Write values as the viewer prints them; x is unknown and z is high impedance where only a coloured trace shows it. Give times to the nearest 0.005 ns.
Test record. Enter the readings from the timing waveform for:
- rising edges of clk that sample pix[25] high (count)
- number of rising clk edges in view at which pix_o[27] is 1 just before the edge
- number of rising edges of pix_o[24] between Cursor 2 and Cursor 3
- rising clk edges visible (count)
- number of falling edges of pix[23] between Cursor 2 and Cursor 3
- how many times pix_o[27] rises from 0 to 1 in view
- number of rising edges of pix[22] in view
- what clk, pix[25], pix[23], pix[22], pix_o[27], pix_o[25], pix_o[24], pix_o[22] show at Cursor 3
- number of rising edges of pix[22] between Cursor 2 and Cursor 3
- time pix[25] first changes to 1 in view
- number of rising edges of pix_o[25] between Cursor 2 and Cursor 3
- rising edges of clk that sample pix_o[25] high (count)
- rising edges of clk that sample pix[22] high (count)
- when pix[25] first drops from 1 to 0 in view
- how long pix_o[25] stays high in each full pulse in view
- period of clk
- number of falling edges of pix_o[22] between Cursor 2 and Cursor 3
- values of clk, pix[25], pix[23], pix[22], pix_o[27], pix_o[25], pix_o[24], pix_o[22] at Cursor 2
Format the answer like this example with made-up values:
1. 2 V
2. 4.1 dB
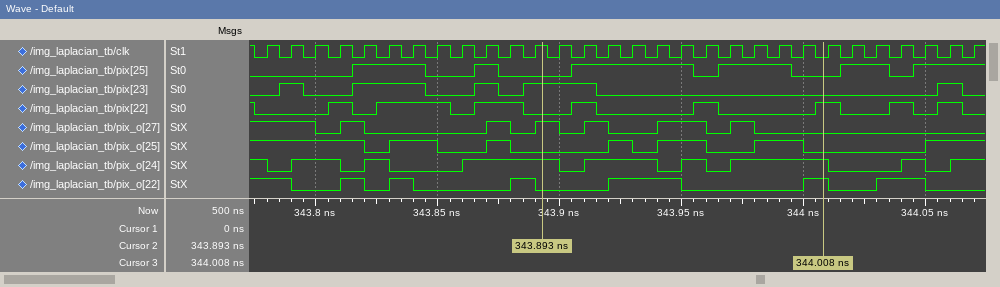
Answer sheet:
1. 17
2. 10
3. 3
4. 30
5. 1
6. 6
7. 8
8. clk=0, pix[25]=0, pix[23]=0, pix[22]=1, pix_o[27]=0, pix_o[25]=0, pix_o[24]=1, pix_o[22]=1
9. 3
10. 343.815 ns
11. 3
12. 15
13. 11
14. 343.845 ns
15. 0.02 ns, 0.01 ns, 0.01 ns, 0.02 ns, 0.02 ns
16. 0.01 ns
17. 1
18. clk=1, pix[25]=0, pix[23]=1, pix[22]=0, pix_o[27]=1, pix_o[25]=0, pix_o[24]=1, pix_o[22]=0
